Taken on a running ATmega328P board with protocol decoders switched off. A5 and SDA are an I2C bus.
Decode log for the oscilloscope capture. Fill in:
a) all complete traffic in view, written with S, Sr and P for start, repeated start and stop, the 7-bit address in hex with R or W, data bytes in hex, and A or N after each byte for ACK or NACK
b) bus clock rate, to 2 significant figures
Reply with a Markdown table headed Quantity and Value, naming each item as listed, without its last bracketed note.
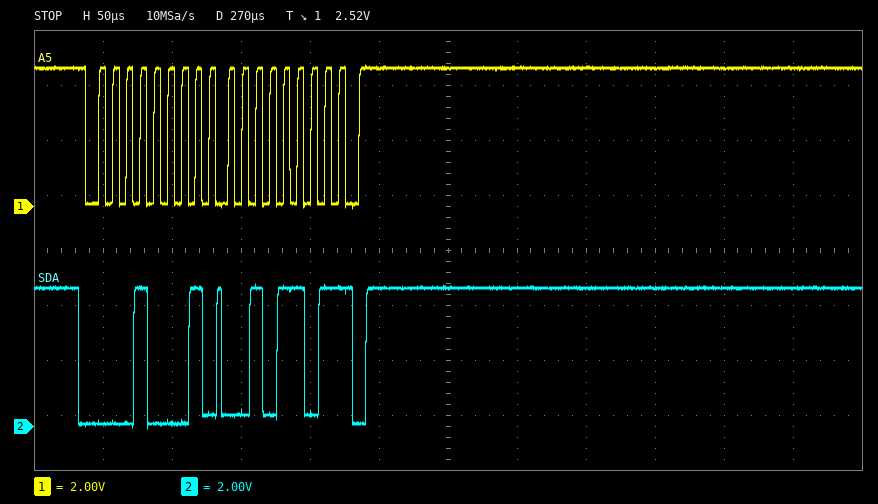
| Quantity | Value |
|---|---|
| all complete traffic in view, written with S, Sr and P for start, repeated start and stop, the 7-bit address in hex with R or W, data bytes in hex, and A or N after each byte for ACK or NACK | S 08R A 2D N P |
| bus clock rate, to 2 significant figures | 100 kHz |
